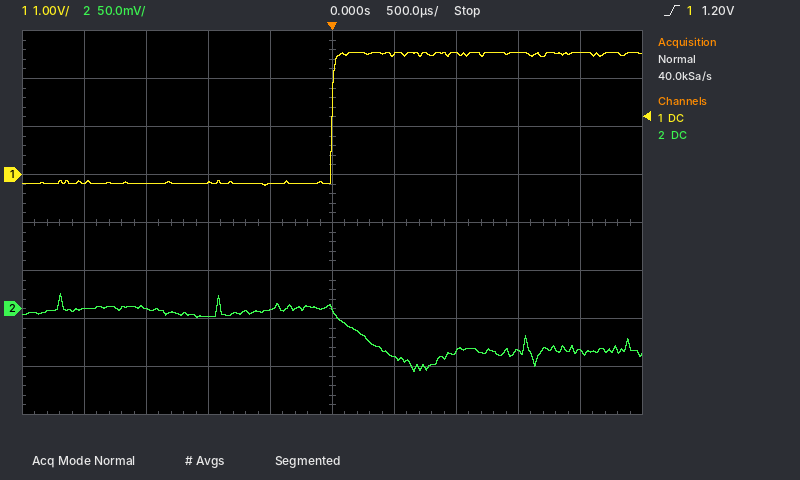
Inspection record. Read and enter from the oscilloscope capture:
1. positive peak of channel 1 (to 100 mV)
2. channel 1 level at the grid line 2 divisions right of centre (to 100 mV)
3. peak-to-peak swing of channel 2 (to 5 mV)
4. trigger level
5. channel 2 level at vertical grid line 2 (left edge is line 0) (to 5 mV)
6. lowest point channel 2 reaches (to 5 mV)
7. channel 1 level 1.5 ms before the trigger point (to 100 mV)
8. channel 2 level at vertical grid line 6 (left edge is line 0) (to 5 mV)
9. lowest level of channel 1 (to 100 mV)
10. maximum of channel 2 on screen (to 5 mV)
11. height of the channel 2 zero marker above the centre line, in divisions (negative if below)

2.5 V
2.5 V
80 mV
1.20 V
0 mV
-65 mV
-200 mV
-50 mV
-200 mV
15 mV
-1.8 div
